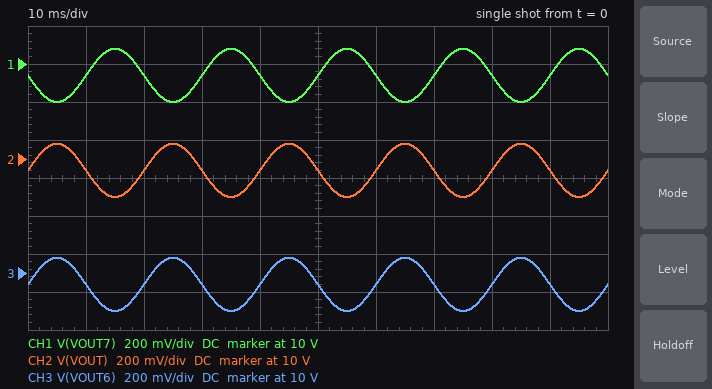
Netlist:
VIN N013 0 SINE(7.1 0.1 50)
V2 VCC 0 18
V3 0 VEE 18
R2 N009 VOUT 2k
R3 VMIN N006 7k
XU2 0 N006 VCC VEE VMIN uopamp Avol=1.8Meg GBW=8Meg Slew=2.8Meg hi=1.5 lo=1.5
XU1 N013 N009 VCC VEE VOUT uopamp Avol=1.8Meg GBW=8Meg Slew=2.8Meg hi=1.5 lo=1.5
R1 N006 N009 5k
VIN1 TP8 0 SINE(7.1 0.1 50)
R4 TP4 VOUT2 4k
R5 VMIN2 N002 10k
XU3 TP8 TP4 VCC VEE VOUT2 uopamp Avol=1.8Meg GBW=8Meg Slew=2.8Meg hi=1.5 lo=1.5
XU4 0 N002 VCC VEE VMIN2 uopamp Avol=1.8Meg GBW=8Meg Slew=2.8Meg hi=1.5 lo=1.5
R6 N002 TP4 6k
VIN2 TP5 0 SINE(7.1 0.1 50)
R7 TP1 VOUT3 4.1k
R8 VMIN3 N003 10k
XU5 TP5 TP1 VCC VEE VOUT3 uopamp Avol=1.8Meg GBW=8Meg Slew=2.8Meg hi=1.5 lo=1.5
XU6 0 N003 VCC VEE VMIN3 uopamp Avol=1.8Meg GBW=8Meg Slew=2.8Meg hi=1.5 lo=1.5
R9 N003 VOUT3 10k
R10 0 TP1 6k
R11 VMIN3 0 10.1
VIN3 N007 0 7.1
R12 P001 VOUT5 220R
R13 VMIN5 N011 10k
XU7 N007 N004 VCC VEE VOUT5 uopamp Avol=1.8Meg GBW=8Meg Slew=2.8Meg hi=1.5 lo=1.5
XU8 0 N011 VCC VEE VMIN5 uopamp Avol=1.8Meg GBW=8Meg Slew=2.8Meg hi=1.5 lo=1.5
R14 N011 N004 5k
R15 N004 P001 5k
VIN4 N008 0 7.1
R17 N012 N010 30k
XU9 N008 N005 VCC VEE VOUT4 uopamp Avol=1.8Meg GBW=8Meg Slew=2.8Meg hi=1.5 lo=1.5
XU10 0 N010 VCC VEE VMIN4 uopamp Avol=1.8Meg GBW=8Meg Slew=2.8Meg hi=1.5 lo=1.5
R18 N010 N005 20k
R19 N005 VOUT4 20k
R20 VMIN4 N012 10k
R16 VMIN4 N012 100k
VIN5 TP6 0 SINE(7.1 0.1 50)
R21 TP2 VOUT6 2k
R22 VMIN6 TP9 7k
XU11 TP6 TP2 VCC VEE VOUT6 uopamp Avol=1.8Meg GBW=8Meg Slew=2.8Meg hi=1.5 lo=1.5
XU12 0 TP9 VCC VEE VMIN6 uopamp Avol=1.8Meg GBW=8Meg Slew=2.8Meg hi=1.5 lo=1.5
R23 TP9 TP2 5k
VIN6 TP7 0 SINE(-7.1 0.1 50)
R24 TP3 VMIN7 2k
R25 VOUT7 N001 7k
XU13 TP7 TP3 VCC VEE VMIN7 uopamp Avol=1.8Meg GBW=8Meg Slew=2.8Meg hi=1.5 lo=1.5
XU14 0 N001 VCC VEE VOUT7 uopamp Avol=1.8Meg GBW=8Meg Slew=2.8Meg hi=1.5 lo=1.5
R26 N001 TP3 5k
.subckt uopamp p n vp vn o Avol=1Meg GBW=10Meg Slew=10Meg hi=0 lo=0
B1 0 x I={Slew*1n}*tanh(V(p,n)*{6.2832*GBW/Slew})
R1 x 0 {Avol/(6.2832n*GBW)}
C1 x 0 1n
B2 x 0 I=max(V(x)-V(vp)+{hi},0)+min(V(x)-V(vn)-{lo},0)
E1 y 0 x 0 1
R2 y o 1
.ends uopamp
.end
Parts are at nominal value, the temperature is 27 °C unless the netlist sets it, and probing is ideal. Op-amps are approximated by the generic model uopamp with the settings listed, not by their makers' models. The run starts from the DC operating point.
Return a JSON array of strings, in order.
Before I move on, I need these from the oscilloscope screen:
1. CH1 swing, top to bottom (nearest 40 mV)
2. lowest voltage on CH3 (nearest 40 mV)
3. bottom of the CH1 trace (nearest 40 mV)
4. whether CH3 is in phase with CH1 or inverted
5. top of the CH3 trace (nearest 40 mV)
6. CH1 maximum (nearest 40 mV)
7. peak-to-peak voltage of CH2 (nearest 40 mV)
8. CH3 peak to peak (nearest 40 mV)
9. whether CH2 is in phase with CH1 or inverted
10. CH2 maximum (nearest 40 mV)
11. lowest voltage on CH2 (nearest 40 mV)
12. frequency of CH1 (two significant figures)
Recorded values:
["280 mV", "9.80 V", "9.80 V", "inverted", "10.08 V", "10.08 V", "280 mV", "280 mV", "inverted", "10.08 V", "9.80 V", "50 Hz"]
